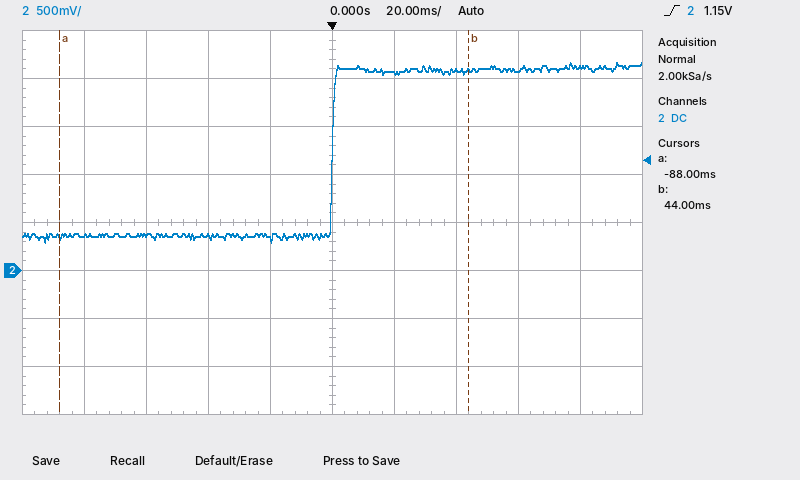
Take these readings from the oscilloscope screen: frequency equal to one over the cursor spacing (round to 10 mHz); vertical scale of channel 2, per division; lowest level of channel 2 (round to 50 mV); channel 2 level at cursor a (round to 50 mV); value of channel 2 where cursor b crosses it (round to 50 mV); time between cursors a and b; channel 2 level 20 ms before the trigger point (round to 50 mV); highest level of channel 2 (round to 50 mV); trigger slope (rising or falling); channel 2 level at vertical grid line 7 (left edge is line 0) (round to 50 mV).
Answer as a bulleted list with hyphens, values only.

- 7.58 Hz
- 500 mV
- 300 mV
- 350 mV
- 2.10 V
- 132 ms
- 350 mV
- 2.15 V
- rising
- 2.10 V
